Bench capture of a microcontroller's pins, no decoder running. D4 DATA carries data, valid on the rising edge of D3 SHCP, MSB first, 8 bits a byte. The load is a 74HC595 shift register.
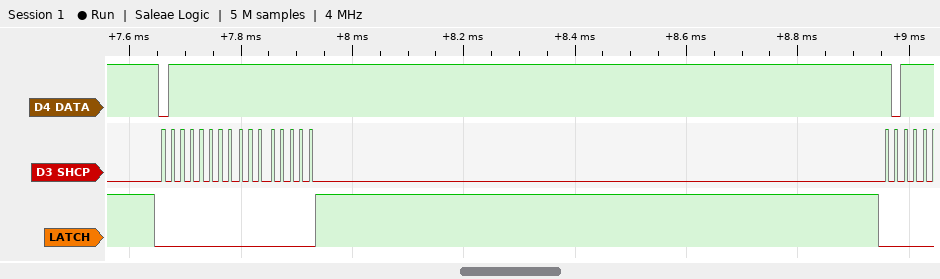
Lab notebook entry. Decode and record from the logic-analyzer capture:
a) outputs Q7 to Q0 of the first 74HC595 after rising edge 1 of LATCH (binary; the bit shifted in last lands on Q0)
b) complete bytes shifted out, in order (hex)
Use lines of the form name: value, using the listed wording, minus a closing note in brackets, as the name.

outputs Q7 to Q0 of the first 74HC595 after rising edge 1 of LATCH: 11111111
complete bytes shifted out, in order: 7F FF
